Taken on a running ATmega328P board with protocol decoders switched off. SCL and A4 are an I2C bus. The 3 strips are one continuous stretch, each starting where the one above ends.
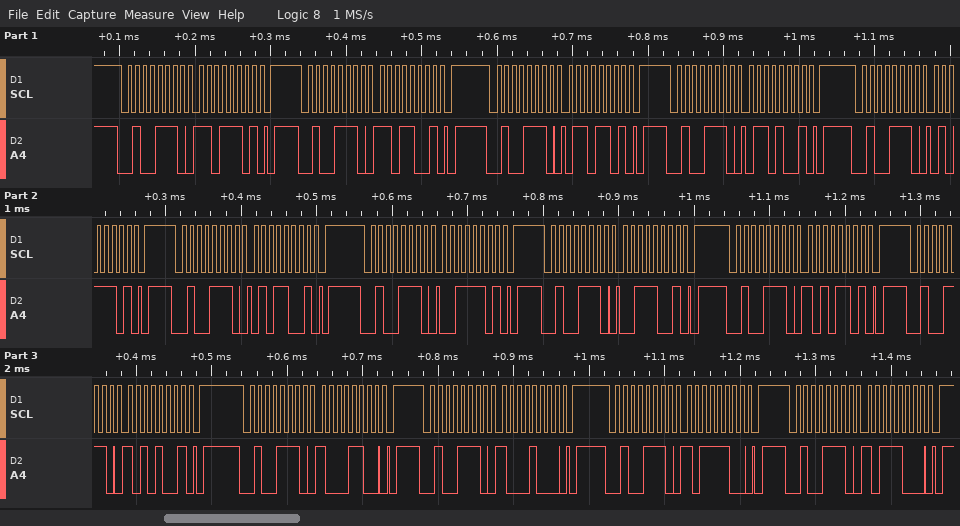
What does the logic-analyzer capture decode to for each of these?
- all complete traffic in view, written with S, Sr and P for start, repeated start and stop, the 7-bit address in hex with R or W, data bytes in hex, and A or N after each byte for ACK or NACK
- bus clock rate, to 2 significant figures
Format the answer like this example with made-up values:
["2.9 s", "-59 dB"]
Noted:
["S 27W A DD A P S 27W A D9 A P S 27W A 6D A P S 27W A 69 A P S 27W A 5D A P S 27W A 59 A P S 27W A 3D A P S 27W A 39 A P S 27W A AD A P S 27W A A9 A P S 27W A 8C A P S 27W A 88 A P S 27W A BC A P S 27W A B8 A P", "100 kHz"]
